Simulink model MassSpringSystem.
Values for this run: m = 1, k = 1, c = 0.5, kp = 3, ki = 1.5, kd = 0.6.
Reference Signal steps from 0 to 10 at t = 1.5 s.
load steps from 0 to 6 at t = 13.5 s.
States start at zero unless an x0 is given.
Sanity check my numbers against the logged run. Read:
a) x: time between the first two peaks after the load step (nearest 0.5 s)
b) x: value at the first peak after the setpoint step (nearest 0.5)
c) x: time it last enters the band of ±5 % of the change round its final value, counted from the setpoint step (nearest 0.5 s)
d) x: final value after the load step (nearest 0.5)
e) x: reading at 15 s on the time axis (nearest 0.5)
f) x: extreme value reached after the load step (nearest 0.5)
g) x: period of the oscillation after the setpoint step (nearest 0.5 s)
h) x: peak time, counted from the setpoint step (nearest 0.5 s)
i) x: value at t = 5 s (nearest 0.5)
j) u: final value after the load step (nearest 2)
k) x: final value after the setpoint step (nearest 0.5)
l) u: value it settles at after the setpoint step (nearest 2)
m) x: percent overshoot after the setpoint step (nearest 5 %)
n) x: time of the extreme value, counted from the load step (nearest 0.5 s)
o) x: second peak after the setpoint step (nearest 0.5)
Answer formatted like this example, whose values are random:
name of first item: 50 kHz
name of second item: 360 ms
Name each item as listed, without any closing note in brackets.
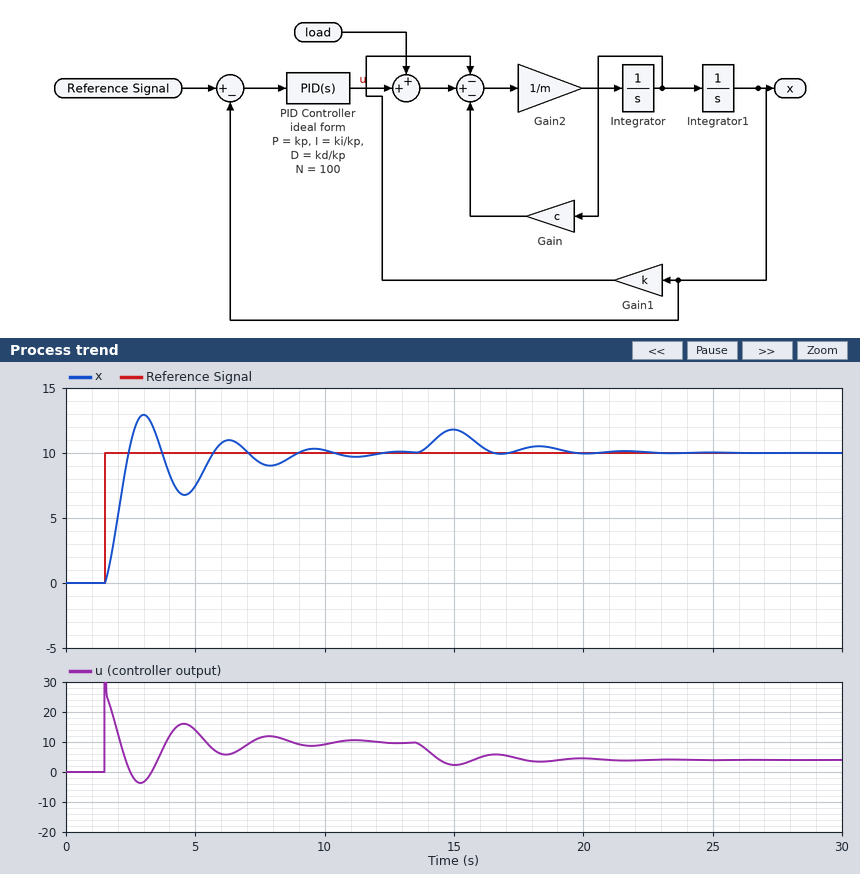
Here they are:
x: time between the first two peaks after the load step: 3.5 s
x: value at the first peak after the setpoint step: 13.0
x: time it last enters the band of ±5 % of the change round its final value, counted from the setpoint step: 7.0 s
x: final value after the load step: 10.0
x: reading at 15 s on the time axis: 12.0
x: extreme value reached after the load step: 12.0
x: period of the oscillation after the setpoint step: 3.5 s
x: peak time, counted from the setpoint step: 1.5 s
x: value at t = 5 s: 7.5
u: final value after the load step: 4
x: final value after the setpoint step: 10.0
u: value it settles at after the setpoint step: 10
x: percent overshoot after the setpoint step: 30 %
x: time of the extreme value, counted from the load step: 1.5 s
x: second peak after the setpoint step: 11.0
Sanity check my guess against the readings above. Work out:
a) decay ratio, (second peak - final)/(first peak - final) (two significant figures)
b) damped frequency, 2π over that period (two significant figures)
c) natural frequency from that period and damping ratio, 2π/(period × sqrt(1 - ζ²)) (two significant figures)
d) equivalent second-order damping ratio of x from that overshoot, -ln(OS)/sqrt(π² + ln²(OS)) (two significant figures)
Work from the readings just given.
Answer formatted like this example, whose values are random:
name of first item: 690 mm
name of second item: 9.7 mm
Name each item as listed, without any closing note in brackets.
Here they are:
decay ratio, (second peak - final)/(first peak - final): 0.33
damped frequency, 2π over that period: 1.8 rad/s
natural frequency from that period and damping ratio, 2π/(period × sqrt(1 - ζ²)): 1.9 rad/s
equivalent second-order damping ratio of x from that overshoot, -ln(OS)/sqrt(π² + ln²(OS)): 0.36
